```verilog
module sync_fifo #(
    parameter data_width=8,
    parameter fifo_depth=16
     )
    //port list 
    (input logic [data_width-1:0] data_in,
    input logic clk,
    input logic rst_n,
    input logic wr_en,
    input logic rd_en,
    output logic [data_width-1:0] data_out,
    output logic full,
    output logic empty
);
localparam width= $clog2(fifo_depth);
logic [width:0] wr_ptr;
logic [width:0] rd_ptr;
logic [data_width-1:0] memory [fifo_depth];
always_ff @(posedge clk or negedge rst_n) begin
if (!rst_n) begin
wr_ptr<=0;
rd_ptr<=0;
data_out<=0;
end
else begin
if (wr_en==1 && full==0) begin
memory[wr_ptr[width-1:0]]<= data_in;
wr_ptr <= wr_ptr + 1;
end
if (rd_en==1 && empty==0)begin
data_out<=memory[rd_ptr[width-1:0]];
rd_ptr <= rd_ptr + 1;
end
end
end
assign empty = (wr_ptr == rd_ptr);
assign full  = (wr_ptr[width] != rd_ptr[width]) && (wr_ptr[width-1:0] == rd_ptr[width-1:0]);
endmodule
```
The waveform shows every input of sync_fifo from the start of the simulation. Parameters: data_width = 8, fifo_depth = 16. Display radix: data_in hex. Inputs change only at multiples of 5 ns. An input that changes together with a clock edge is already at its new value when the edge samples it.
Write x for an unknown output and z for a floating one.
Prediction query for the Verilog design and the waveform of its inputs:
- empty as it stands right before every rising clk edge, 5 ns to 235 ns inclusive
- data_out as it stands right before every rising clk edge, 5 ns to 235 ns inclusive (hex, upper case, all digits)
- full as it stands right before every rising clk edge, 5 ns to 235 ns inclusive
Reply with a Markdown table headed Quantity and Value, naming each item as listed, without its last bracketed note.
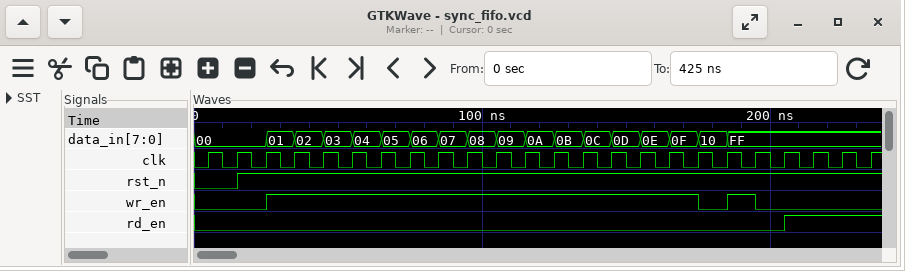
| Quantity | Value |
|---|---|
| empty as it stands right before every rising clk edge, 5 ns to 235 ns inclusive | 1 1 1 0 0 0 0 0 0 0 0 0 0 0 0 0 0 0 0 0 0 0 0 0 |
| data_out as it stands right before every rising clk edge, 5 ns to 235 ns inclusive | 00, 00, 00, 00, 00, 00, 00, 00, 00, 00, 00, 00, 00, 00, 00, 00, 00, 00, 00, 00, 00, 01, 02, 03 |
| full as it stands right before every rising clk edge, 5 ns to 235 ns inclusive | 0 0 0 0 0 0 0 0 0 0 0 0 0 0 0 0 0 0 0 1 1 0 0 0 |
